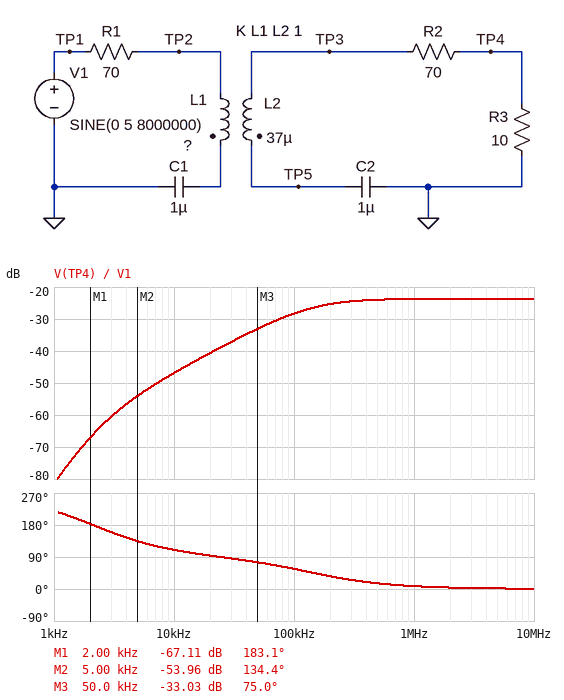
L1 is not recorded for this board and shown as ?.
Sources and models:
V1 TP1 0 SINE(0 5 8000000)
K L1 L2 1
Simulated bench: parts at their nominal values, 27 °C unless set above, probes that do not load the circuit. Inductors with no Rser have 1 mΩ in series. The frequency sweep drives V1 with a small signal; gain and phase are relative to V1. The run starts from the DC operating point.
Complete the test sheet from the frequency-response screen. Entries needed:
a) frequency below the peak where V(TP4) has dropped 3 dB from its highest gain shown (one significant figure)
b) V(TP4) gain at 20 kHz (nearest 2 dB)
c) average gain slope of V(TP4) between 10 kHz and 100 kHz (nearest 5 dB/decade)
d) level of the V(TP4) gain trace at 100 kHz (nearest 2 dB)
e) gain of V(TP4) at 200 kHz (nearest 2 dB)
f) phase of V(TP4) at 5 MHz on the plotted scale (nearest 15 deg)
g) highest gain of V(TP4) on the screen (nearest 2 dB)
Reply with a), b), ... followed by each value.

a) 100 kHz
b) -40 dB
c) 20 dB/decade
d) -28 dB
e) -26 dB
f) 0 deg
g) -24 dB
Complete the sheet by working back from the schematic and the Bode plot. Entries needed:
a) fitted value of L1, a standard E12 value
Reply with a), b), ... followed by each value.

a) 47 µH
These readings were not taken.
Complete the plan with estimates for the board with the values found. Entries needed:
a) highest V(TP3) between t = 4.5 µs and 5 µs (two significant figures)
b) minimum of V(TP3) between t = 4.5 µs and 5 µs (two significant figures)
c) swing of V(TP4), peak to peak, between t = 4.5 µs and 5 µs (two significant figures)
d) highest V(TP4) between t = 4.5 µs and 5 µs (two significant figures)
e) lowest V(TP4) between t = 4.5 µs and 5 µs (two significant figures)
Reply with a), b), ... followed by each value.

a) 2.6 V
b) -2.6 V
c) 660 mV
d) 330 mV
e) -330 mV
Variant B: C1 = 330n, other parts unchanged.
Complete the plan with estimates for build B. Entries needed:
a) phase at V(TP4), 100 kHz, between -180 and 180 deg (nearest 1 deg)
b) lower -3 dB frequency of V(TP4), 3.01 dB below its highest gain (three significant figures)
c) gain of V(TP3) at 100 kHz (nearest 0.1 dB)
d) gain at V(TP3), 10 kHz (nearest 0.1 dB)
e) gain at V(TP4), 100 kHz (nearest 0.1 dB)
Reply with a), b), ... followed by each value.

a) 59 deg
b) 136 kHz
c) -10.1 dB
d) -30.2 dB
e) -28.2 dB
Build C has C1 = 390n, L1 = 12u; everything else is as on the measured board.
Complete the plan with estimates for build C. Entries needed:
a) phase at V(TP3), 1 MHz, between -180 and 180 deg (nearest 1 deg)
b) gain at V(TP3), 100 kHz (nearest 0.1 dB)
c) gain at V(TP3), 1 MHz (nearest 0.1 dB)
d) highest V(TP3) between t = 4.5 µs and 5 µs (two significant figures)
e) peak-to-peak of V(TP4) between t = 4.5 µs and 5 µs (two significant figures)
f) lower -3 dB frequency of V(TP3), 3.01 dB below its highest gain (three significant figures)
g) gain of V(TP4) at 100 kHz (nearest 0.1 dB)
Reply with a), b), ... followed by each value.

a) 14 deg
b) -15.0 dB
c) -6.7 dB
d) 2.4 V
e) 590 mV
f) 248 kHz
g) -33.1 dB
